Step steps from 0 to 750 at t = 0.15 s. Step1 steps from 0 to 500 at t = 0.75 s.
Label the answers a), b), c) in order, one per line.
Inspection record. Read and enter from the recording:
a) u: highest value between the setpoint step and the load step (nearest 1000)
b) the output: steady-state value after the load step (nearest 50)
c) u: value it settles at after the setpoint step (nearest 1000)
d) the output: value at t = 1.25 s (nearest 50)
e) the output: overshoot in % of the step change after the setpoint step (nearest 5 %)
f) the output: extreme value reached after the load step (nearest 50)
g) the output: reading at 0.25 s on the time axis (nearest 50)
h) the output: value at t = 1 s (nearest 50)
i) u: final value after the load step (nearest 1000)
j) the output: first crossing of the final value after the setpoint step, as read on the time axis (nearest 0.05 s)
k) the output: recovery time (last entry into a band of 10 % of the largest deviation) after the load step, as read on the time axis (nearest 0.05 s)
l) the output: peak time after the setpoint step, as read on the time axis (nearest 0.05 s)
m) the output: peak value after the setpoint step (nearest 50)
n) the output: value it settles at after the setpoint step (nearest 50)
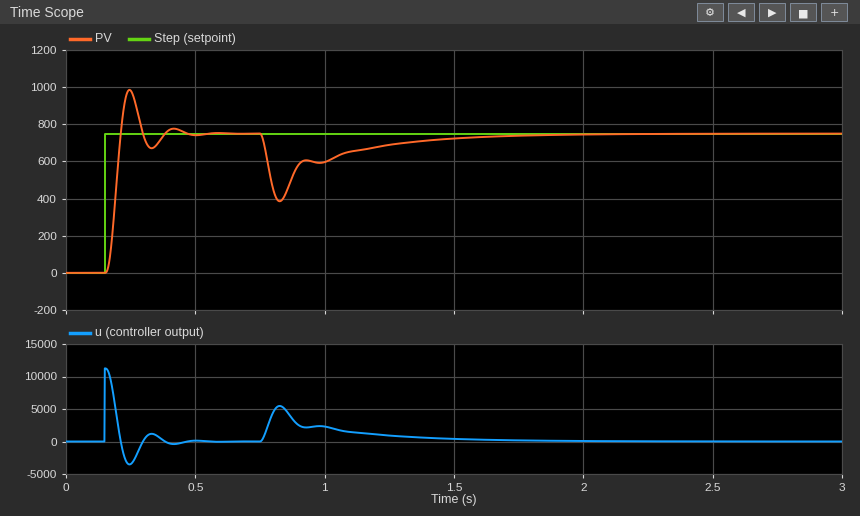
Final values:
a) 11000
b) 750
c) 0
d) 700
e) 30 %
f) 400
g) 1000
h) 600
i) 0
j) 0.20 s
k) 1.40 s
l) 0.25 s
m) 1000
n) 750
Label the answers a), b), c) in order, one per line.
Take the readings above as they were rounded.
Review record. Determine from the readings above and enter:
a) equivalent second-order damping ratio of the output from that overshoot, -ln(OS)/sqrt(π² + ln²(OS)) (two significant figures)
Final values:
a) 0.36
